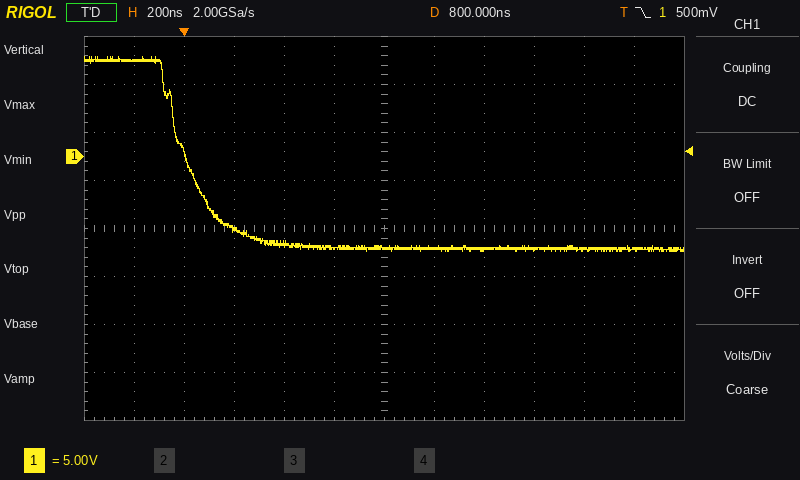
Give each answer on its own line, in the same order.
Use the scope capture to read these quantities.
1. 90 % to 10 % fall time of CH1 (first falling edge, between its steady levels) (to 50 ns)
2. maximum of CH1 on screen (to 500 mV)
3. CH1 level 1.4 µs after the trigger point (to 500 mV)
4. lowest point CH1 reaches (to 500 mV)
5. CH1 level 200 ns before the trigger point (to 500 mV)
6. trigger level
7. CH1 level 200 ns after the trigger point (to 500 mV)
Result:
300 ns
10.5 V
-9.5 V
-10.0 V
10.0 V
500 mV
-7.5 V
